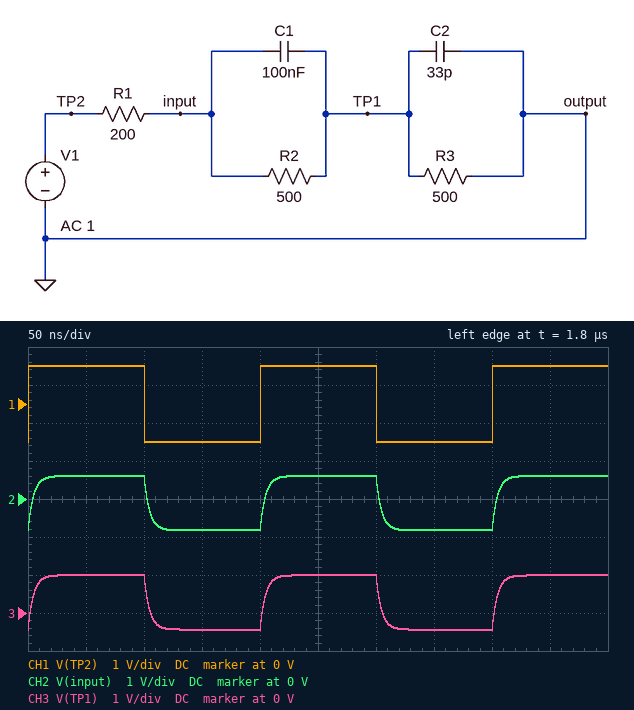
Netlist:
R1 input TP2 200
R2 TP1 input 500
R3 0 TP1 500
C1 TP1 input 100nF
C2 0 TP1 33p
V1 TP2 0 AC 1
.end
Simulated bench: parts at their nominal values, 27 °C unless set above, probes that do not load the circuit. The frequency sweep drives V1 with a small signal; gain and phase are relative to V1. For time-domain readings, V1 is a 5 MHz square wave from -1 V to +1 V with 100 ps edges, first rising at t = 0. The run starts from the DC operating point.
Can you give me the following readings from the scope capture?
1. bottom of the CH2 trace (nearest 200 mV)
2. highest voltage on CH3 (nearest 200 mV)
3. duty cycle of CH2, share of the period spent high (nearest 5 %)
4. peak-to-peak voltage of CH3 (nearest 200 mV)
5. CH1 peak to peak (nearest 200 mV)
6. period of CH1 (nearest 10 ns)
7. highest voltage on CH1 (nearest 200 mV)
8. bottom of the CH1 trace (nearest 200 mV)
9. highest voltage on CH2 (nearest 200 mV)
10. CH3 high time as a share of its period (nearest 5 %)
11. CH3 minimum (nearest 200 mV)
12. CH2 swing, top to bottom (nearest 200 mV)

-800 mV
1.0 V
50 %
1.4 V
2.0 V
200 ns
1.0 V
-1.0 V
600 mV
50 %
-400 mV
1.4 V
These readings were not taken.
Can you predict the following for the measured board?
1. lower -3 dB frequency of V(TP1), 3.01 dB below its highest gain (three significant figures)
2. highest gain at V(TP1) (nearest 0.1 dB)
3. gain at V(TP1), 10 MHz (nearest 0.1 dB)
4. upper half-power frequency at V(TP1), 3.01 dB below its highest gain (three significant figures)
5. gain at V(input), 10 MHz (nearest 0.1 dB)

3.08 kHz
-2.9 dB
-3.3 dB
33.8 MHz
-3.3 dB
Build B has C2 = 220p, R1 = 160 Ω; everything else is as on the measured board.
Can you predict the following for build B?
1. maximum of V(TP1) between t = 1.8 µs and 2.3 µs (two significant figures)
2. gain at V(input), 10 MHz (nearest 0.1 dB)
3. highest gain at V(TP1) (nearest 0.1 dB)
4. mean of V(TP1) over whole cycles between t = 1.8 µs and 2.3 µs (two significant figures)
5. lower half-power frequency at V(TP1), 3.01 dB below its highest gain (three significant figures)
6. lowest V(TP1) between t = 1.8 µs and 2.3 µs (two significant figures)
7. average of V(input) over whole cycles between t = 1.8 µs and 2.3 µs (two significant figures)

1.0 V
-8.2 dB
-2.4 dB
300 mV
3.30 kHz
-420 mV
-97 mV
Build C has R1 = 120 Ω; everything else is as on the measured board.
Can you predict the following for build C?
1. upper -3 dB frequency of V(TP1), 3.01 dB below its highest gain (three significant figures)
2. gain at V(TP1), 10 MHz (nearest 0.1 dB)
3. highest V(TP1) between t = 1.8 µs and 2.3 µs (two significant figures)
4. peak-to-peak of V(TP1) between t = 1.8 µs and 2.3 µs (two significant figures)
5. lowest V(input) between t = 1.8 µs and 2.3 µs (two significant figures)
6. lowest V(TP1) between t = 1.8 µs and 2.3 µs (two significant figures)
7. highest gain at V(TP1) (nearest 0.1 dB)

49.9 MHz
-2.0 dB
1.1 V
1.6 V
-890 mV
-470 mV
-1.9 dB
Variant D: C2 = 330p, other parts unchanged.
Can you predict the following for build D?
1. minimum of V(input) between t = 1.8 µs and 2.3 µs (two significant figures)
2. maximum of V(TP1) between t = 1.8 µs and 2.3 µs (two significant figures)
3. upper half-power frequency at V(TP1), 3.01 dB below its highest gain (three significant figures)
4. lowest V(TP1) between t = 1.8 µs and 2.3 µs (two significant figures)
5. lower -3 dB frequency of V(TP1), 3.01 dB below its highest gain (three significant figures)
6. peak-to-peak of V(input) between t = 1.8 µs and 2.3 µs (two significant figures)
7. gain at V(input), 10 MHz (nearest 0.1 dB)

-670 mV
840 mV
3.39 MHz
-290 mV
3.05 kHz
1.1 V
-12.8 dB
